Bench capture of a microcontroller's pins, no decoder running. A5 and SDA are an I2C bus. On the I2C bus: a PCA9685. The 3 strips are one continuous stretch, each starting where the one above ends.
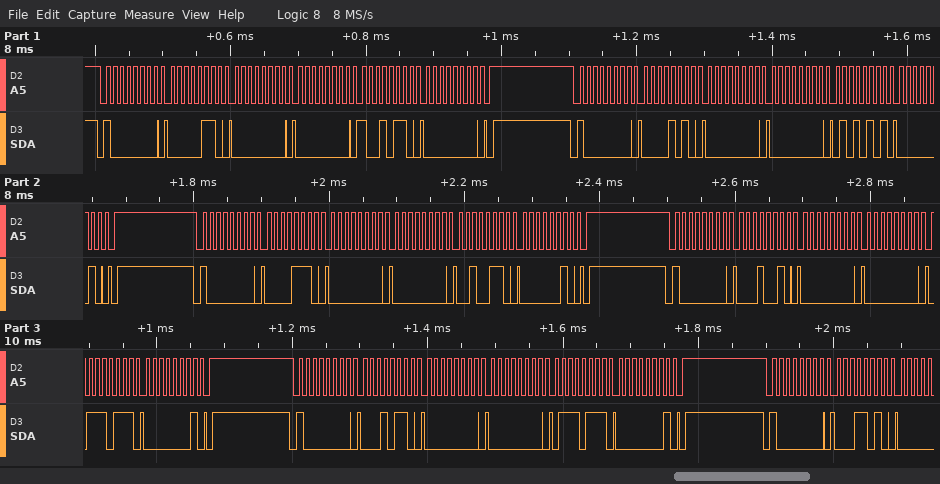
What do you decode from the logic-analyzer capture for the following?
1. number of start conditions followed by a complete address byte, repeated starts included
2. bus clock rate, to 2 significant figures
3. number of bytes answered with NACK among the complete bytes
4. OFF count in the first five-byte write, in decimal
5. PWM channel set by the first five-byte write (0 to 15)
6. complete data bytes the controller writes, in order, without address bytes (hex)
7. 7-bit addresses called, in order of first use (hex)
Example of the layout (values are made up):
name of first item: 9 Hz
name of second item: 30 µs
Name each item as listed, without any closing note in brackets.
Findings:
number of start conditions followed by a complete address byte, repeated starts included: 6
bus clock rate, to 2 significant figures: 100 kHz
number of bytes answered with NACK among the complete bytes: 0
OFF count in the first five-byte write, in decimal: 150
PWM channel set by the first five-byte write: 0
complete data bytes the controller writes, in order, without address bytes: 06 00 00 96 00 0A 00 00 55 02 0E 00 00 26 02 12 00 00 77 01 16 00 00 77 01 1A
7-bit addresses called, in order of first use: 0x40
